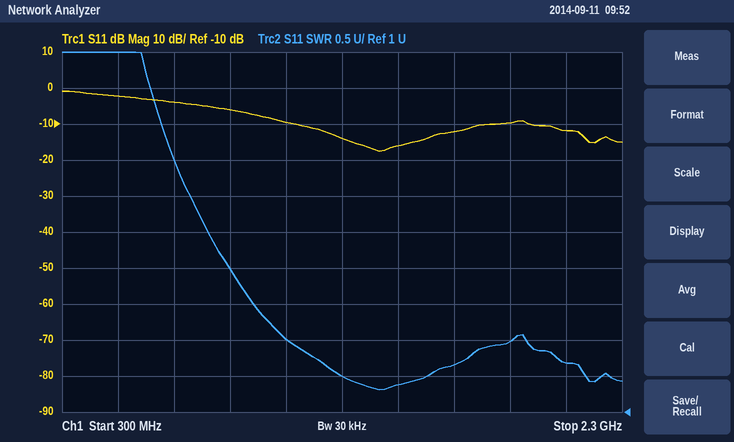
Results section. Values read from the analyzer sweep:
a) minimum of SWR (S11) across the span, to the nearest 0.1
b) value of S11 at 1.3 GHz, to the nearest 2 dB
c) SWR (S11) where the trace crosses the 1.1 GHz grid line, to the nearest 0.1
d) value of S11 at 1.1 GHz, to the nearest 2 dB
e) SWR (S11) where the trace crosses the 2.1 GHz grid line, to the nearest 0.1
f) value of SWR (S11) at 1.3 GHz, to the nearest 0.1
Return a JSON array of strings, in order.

["1.3", "-14 dB", "2.0", "-10 dB", "1.7", "1.5"]
